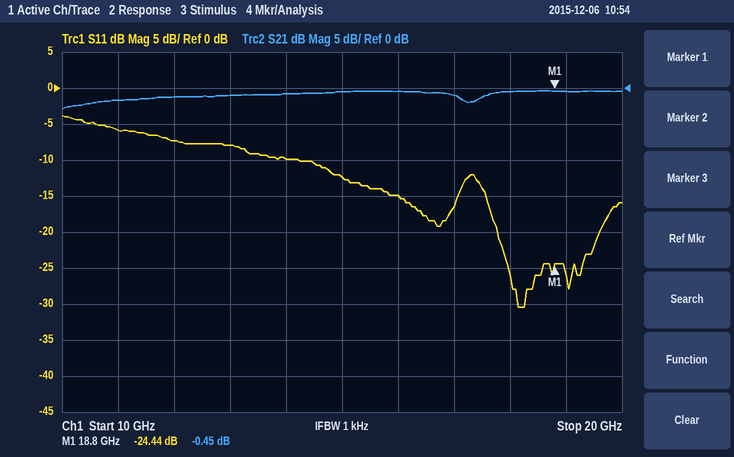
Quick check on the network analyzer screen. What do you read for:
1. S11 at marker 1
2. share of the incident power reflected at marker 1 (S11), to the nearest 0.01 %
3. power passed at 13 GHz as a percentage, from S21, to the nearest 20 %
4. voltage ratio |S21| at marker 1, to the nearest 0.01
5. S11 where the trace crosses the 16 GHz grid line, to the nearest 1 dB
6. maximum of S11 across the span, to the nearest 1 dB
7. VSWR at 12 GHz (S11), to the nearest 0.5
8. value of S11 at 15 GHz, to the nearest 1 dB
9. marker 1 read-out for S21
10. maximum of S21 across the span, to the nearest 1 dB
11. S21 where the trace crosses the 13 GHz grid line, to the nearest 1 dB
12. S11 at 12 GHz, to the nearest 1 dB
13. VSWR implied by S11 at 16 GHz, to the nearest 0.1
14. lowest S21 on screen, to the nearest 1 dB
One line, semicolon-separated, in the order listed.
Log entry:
-24.44 dB; 0.36 %; 80 %; 0.95; -15 dB; -4 dB; 2.5; -12 dB; -0.45 dB; 0 dB; -1 dB; -7 dB; 1.4; -3 dB
